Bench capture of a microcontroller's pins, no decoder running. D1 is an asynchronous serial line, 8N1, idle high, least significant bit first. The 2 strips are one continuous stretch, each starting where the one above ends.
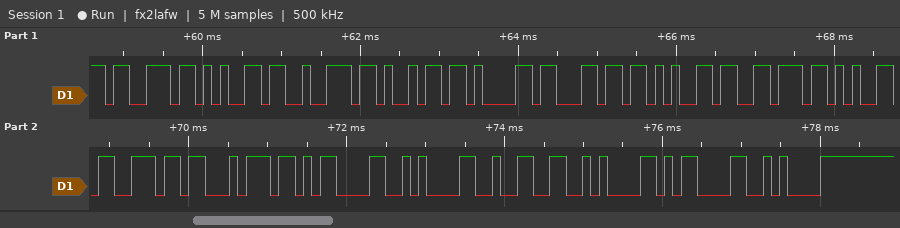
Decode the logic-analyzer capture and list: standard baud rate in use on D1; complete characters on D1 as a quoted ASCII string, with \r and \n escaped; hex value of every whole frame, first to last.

9600 baud
"serialevent\r\n2\n\r\n"
73 65 72 69 61 6C 65 76 65 6E 74 0D 0A 32 0A 0D 0A
